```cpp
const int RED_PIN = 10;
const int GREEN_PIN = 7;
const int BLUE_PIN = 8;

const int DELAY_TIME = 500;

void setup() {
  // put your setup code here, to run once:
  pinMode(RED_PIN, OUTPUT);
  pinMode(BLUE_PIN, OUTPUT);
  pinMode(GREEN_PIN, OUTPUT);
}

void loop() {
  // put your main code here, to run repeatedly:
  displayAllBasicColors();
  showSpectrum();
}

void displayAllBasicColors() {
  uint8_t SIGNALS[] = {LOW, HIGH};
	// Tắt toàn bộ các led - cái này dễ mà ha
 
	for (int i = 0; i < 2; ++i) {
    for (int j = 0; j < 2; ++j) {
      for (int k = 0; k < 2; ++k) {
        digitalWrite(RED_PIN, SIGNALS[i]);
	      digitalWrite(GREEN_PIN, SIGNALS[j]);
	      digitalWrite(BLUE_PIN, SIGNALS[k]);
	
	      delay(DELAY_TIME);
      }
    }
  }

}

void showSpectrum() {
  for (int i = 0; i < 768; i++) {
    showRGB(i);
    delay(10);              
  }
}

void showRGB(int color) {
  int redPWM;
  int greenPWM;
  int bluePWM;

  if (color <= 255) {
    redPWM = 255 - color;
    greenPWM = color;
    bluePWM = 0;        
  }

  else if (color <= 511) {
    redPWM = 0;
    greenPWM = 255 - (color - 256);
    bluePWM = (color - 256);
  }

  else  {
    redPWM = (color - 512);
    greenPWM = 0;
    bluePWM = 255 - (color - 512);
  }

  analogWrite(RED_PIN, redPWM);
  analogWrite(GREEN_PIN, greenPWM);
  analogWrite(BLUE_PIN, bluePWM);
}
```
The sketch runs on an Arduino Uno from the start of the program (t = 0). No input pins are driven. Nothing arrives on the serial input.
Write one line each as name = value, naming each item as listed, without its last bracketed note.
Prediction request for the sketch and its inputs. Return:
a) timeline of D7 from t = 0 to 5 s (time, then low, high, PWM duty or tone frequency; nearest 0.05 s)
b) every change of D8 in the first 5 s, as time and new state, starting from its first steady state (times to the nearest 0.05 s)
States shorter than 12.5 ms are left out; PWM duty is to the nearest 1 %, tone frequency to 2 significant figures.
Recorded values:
timeline of D7 from t = 0 to 5 s = 0 s low; 1 s high; 2 s low; 3 s high; 4 s low
every change of D8 in the first 5 s, as time and new state, starting from its first steady state = 0 s low; 0.5 s high; 1 s low; 1.5 s high; 2 s low; 2.5 s high; 3 s low; 3.5 s high; 4 s low
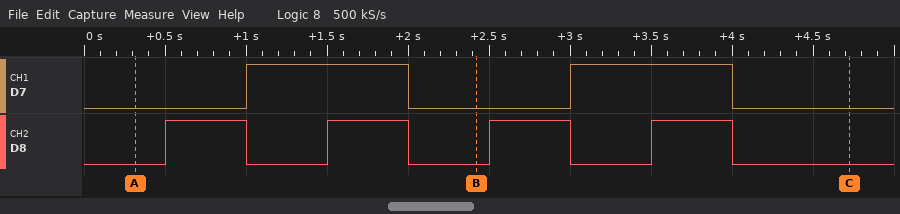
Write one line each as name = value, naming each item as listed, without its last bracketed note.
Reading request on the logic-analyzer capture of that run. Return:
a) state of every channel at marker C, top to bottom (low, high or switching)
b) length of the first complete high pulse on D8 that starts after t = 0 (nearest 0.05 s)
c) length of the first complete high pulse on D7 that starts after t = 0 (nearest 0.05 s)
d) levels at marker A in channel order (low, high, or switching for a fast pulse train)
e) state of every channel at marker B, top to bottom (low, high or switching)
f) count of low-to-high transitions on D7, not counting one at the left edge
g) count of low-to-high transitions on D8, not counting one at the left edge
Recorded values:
state of every channel at marker C, top to bottom = D7 low, D8 low
length of the first complete high pulse on D8 that starts after t = 0 = 0.50 s
length of the first complete high pulse on D7 that starts after t = 0 = 1.00 s
levels at marker A in channel order = D7 low, D8 low
state of every channel at marker B, top to bottom = D7 low, D8 low
count of low-to-high transitions on D7, not counting one at the left edge = 2
count of low-to-high transitions on D8, not counting one at the left edge = 4
